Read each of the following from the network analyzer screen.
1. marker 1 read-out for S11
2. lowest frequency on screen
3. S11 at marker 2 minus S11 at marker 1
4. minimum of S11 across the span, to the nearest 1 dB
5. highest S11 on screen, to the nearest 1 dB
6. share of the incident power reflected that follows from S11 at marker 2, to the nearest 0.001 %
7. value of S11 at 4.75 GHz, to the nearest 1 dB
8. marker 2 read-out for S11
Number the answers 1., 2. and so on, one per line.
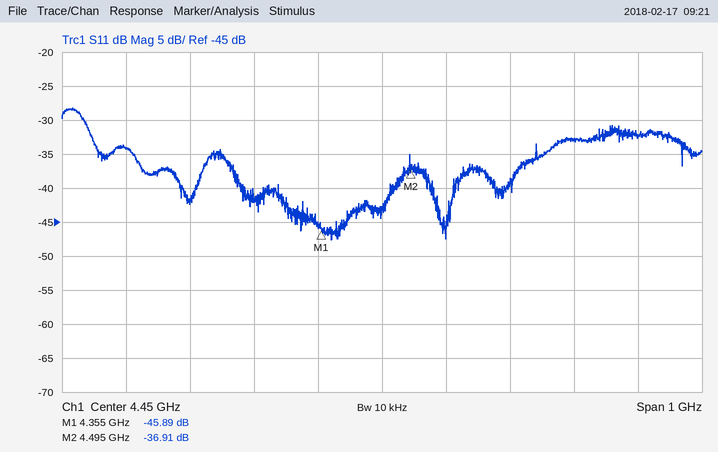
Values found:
1. -45.89 dB
2. 3.95 GHz
3. 8.98 dB
4. -48 dB
5. -28 dB
6. 0.020 %
7. -33 dB
8. -36.91 dB
